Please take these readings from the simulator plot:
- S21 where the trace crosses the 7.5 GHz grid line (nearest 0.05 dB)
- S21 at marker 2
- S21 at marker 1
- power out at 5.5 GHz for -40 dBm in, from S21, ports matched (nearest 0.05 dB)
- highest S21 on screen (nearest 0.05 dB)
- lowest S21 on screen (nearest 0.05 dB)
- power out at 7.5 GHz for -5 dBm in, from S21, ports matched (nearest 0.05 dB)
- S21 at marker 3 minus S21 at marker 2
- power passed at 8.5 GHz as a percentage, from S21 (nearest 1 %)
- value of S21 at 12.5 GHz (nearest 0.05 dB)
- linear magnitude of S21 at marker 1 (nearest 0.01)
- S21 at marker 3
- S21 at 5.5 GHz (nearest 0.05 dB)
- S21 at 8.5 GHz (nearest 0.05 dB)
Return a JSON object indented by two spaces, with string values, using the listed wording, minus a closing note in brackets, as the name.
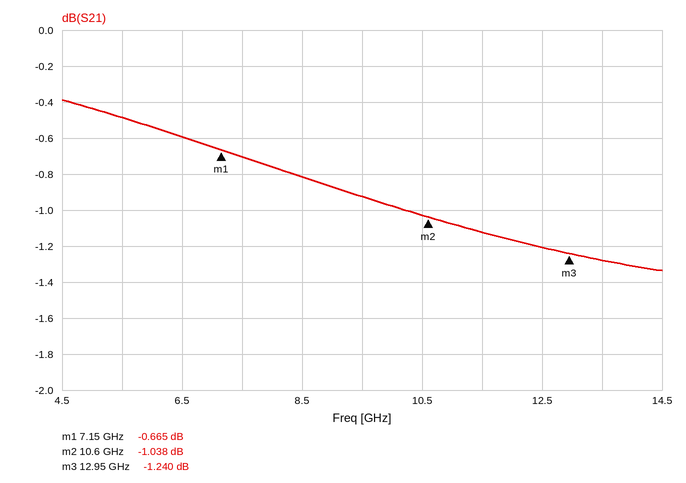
{
  "S21 where the trace crosses the 7.5 GHz grid line": "-0.70 dB",
  "S21 at marker 2": "-1.038 dB",
  "S21 at marker 1": "-0.665 dB",
  "power out at 5.5 GHz for -40 dBm in, from S21, ports matched": "-40.50 dBm",
  "highest S21 on screen": "-0.40 dB",
  "lowest S21 on screen": "-1.35 dB",
  "power out at 7.5 GHz for -5 dBm in, from S21, ports matched": "-5.70 dBm",
  "S21 at marker 3 minus S21 at marker 2": "-0.202 dB",
  "power passed at 8.5 GHz as a percentage, from S21": "83 %",
  "value of S21 at 12.5 GHz": "-1.20 dB",
  "linear magnitude of S21 at marker 1": "0.93",
  "S21 at marker 3": "-1.240 dB",
  "S21 at 5.5 GHz": "-0.50 dB",
  "S21 at 8.5 GHz": "-0.80 dB"
}
